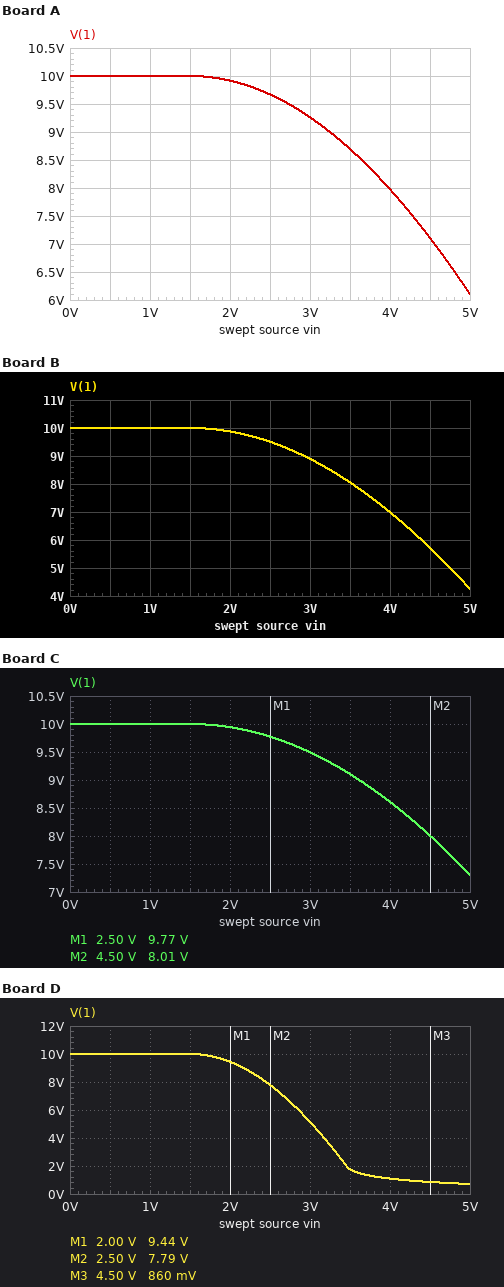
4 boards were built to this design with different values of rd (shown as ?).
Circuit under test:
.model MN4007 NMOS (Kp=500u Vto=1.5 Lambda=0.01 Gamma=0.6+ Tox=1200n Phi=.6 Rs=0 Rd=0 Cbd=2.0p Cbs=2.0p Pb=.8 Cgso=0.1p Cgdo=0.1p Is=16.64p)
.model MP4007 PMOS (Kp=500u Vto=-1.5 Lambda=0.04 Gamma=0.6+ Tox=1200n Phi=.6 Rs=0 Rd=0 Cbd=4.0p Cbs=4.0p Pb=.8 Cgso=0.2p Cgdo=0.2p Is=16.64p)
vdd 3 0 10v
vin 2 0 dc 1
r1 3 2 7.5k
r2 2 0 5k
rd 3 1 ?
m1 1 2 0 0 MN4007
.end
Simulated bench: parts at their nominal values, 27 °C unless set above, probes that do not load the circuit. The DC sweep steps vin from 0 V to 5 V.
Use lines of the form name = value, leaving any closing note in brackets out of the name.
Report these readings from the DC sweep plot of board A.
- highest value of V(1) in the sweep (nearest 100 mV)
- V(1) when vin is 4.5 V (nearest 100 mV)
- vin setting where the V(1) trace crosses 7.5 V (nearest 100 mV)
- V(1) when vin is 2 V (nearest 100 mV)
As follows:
highest value of V(1) in the sweep = 10.0 V
V(1) when vin is 4.5 V = 7.1 V
vin setting where the V(1) trace crosses 7.5 V = 4.3 V
V(1) when vin is 2 V = 9.9 V
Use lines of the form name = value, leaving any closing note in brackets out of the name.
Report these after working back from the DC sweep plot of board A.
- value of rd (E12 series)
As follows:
value of rd = 1.2 kΩ
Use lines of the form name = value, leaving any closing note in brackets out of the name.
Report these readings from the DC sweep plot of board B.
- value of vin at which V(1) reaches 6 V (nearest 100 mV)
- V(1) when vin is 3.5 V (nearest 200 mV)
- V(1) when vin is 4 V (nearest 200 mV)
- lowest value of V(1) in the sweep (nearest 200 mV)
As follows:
value of vin at which V(1) reaches 6 V = 4.4 V
V(1) when vin is 3.5 V = 8.0 V
V(1) when vin is 4 V = 7.0 V
lowest value of V(1) in the sweep = 4.2 V
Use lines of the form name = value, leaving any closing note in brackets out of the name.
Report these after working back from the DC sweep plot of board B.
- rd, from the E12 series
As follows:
rd, from the E12 series = 1.8 kΩ
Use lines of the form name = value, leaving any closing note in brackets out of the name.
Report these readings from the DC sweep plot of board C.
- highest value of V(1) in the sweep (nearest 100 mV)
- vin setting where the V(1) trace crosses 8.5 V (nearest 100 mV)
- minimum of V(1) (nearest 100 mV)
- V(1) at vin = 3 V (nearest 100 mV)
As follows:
highest value of V(1) in the sweep = 10.0 V
vin setting where the V(1) trace crosses 8.5 V = 4.1 V
minimum of V(1) = 7.3 V
V(1) at vin = 3 V = 9.5 V
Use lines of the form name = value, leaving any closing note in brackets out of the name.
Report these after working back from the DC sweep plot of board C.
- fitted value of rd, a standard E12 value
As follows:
fitted value of rd, a standard E12 value = 820 Ω
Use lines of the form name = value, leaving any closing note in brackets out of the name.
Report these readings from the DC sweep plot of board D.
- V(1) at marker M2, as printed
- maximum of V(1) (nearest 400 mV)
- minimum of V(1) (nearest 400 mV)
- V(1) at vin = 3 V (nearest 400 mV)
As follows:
V(1) at marker M2, as printed = 7.79 V
maximum of V(1) = 10.0 V
minimum of V(1) = 800 mV
V(1) at vin = 3 V = 5.2 V
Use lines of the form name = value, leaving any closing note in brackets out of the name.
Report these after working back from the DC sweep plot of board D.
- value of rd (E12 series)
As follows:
value of rd = 8.2 kΩ
